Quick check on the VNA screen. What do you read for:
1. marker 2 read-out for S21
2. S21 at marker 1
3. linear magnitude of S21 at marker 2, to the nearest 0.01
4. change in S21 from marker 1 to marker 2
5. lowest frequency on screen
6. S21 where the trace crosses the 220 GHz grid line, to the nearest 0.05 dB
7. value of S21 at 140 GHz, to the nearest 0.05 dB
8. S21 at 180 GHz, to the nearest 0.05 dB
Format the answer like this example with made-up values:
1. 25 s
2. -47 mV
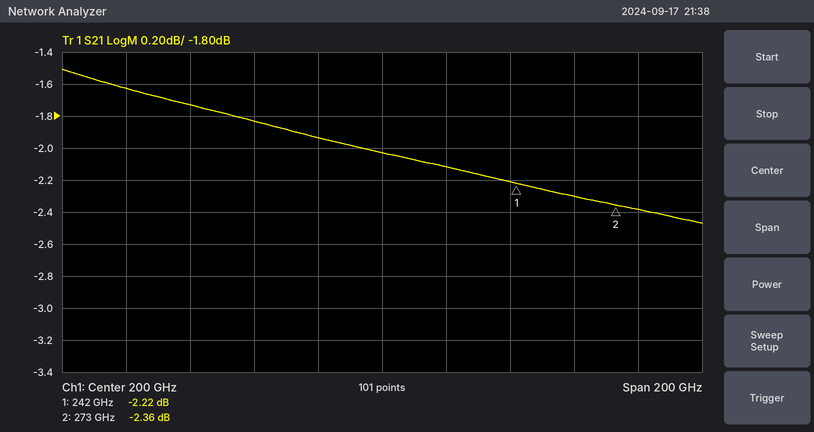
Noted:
1. -2.36 dB
2. -2.22 dB
3. 0.76
4. -0.14 dB
5. 100 GHz
6. -2.10 dB
7. -1.75 dB
8. -1.95 dB
